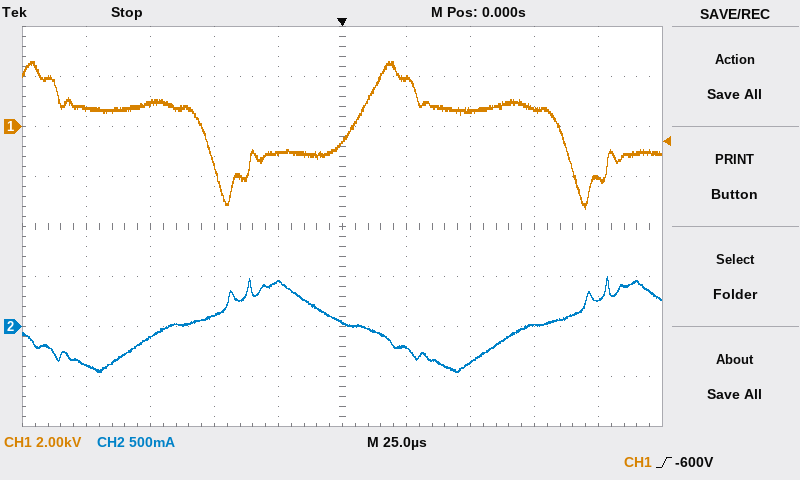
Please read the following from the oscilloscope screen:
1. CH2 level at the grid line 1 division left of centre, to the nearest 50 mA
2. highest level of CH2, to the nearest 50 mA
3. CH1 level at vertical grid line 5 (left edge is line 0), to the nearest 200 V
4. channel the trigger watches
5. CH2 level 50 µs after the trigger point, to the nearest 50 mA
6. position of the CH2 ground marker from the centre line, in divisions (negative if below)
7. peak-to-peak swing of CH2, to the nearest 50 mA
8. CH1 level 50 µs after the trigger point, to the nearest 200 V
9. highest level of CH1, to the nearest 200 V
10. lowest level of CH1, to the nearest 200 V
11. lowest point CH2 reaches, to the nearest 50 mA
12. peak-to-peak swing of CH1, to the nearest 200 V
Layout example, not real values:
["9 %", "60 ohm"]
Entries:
["450 mA", "500 mA", "-600 V", "CH1", "-350 mA", "-2.0 div", "950 mA", "600 V", "2.6 kV", "-3.4 kV", "-450 mA", "6.0 kV"]
